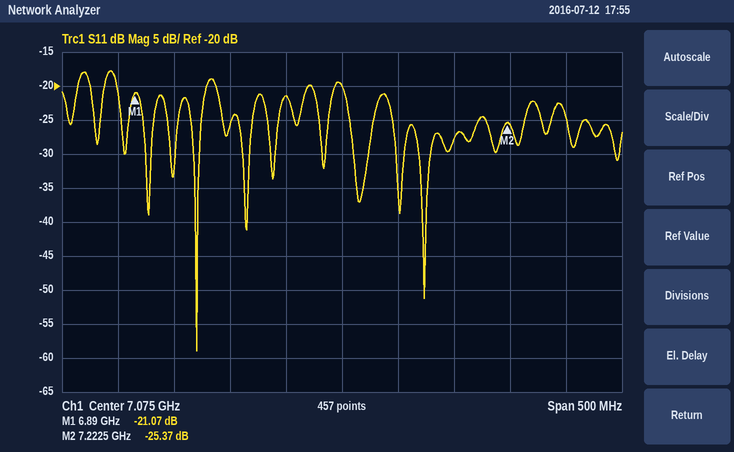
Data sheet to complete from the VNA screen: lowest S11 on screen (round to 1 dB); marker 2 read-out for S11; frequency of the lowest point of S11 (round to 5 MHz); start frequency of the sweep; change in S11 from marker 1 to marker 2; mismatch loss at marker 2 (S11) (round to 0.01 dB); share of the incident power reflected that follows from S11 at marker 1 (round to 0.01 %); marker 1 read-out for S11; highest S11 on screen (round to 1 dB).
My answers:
-59 dB
-25.37 dB
6.945 GHz
6.825 GHz
-4.30 dB
0.01 dB
0.78 %
-21.07 dB
-18 dB
